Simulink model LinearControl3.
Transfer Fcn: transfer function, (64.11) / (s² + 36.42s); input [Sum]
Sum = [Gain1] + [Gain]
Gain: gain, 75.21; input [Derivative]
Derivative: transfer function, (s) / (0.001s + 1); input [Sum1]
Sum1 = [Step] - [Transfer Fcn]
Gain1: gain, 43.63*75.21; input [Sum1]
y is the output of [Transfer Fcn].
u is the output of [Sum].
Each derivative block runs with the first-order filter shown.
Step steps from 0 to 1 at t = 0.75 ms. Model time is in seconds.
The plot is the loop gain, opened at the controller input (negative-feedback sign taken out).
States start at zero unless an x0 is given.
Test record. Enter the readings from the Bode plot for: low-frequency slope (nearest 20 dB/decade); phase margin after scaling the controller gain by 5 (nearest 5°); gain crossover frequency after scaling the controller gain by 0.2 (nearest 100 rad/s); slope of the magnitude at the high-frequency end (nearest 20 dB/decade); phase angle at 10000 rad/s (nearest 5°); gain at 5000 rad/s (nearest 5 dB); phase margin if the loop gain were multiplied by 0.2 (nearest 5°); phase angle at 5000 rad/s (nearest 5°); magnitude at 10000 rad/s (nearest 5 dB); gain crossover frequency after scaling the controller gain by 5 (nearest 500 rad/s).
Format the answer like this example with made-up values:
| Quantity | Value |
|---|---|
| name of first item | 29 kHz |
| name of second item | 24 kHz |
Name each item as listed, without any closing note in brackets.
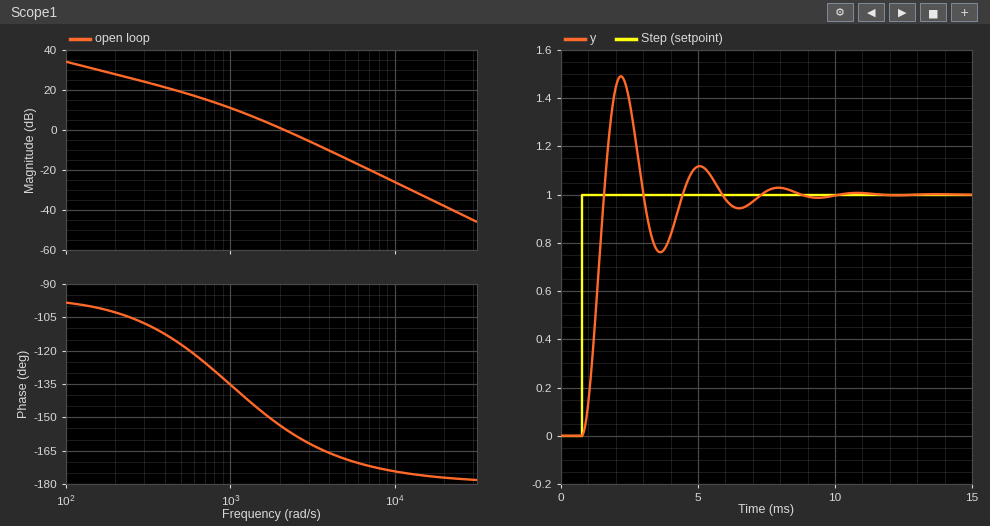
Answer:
| Quantity | Value |
|---|---|
| low-frequency slope | -20 dB/decade |
| phase margin after scaling the controller gain by 5 | 10° |
| gain crossover frequency after scaling the controller gain by 0.2 | 800 rad/s |
| slope of the magnitude at the high-frequency end | -40 dB/decade |
| phase angle at 10000 rad/s | -175° |
| gain at 5000 rad/s | -15 dB |
| phase margin if the loop gain were multiplied by 0.2 | 50° |
| phase angle at 5000 rad/s | -170° |
| magnitude at 10000 rad/s | -25 dB |
| gain crossover frequency after scaling the controller gain by 5 | 5000 rad/s |
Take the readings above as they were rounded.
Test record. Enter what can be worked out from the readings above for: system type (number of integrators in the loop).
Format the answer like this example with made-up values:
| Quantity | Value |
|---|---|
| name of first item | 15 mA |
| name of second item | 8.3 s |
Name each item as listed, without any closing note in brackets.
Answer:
| Quantity | Value |
|---|---|
| system type | 1 |
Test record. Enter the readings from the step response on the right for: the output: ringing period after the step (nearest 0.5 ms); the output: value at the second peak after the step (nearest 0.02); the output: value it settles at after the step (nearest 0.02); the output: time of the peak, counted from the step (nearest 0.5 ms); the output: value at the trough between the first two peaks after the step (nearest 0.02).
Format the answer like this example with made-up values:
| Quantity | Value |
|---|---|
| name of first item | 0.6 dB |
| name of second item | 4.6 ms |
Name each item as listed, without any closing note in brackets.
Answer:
| Quantity | Value |
|---|---|
| the output: ringing period after the step | 3.0 ms |
| the output: value at the second peak after the step | 1.12 |
| the output: value it settles at after the step | 1.00 |
| the output: time of the peak, counted from the step | 1.5 ms |
| the output: value at the trough between the first two peaks after the step | 0.76 |
